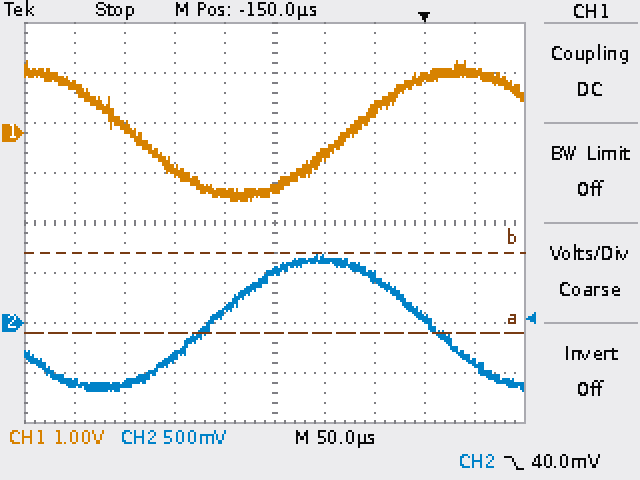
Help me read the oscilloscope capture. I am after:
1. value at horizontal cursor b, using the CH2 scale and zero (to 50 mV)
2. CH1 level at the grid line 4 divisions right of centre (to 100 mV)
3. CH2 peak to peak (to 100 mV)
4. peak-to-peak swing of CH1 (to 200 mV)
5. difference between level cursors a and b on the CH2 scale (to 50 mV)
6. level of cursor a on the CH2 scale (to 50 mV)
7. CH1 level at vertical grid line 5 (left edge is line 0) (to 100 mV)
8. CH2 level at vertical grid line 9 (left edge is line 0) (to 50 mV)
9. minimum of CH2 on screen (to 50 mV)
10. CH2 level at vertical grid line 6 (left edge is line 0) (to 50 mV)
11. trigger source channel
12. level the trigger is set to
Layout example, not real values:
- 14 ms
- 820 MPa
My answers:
- 700 mV
- 1.2 V
- 1.40 V
- 2.8 V
- 800 mV
- -100 mV
- -1.1 V
- -400 mV
- -700 mV
- 650 mV
- CH2
- 40.0 mV
